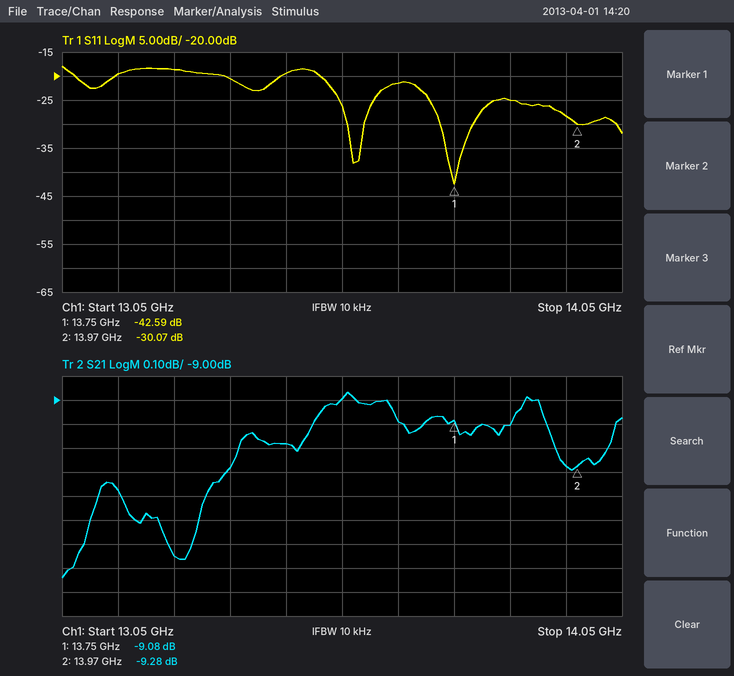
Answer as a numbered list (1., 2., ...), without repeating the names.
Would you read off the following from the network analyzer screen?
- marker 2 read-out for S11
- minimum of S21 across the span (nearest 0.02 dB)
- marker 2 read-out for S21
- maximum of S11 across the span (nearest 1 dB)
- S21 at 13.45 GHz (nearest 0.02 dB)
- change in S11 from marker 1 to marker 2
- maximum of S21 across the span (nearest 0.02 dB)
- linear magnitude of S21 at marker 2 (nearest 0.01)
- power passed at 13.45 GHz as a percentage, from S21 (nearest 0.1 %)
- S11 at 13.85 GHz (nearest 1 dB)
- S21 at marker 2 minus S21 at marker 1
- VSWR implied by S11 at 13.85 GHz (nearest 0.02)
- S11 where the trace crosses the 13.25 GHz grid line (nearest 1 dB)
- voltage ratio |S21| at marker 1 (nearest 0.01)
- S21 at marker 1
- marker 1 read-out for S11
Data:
1. -30.07 dB
2. -9.74 dB
3. -9.28 dB
4. -18 dB
5. -9.18 dB
6. 12.52 dB
7. -8.96 dB
8. 0.34
9. 12.1 %
10. -25 dB
11. -0.20 dB
12. 1.12
13. -19 dB
14. 0.35
15. -9.08 dB
16. -42.59 dB
